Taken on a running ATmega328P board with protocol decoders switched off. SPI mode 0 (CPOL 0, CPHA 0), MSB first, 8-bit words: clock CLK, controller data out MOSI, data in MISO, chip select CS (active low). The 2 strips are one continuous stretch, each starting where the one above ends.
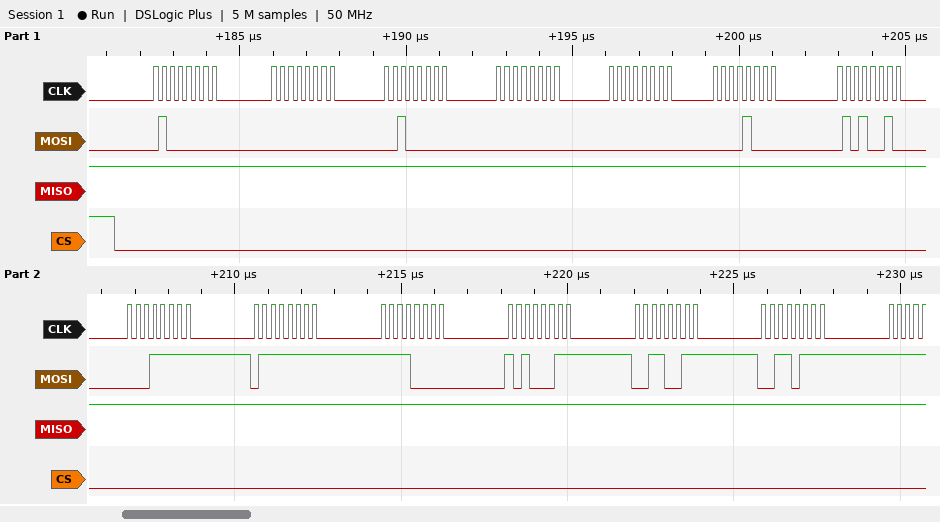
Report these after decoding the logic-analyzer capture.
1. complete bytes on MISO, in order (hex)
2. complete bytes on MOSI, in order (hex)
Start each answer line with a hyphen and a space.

- FF FF FF FF FF FF FF FF FF FF FF FF FF
- 40 00 20 00 00 08 52 1F 7F F0 A3 33 37
